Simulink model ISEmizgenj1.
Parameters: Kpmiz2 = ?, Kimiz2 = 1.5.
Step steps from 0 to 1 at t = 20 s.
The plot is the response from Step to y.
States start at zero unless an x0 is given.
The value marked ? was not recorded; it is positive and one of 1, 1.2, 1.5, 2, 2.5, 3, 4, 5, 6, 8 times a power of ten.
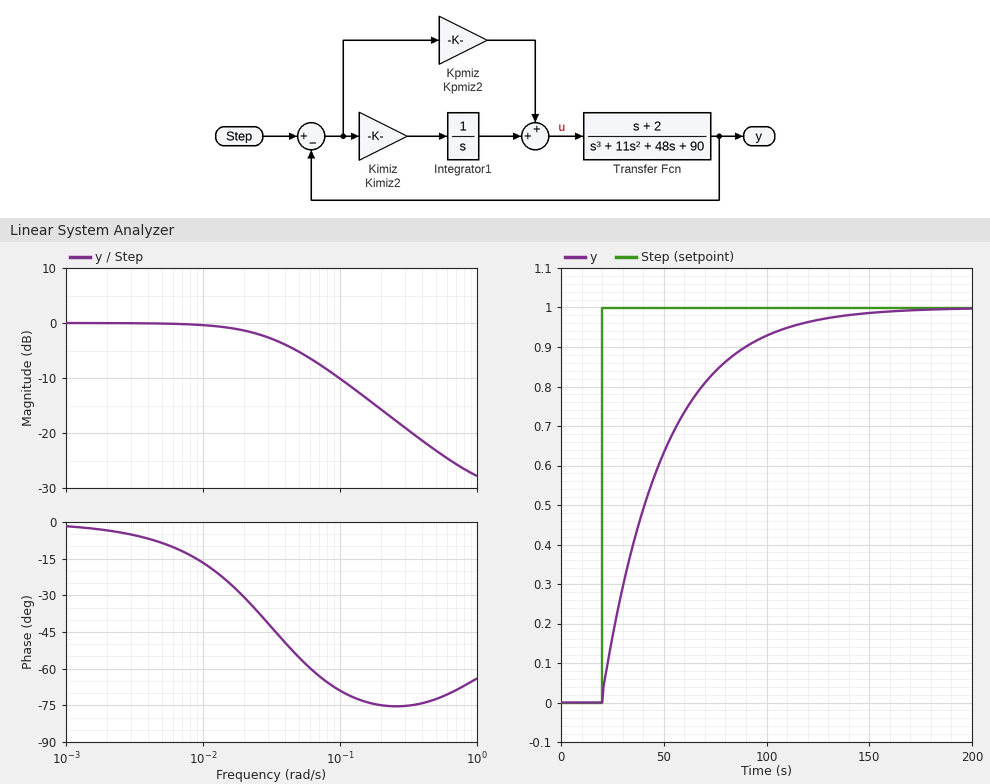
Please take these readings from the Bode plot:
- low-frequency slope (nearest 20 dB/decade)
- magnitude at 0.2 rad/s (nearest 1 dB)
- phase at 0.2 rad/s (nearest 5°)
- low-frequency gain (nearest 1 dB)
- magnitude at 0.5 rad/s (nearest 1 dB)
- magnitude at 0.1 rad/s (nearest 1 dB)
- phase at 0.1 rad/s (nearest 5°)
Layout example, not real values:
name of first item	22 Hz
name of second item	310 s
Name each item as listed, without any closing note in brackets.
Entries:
low-frequency slope	0 dB/decade
magnitude at 0.2 rad/s	-16 dB
phase at 0.2 rad/s	-75°
low-frequency gain	0 dB
magnitude at 0.5 rad/s	-23 dB
magnitude at 0.1 rad/s	-10 dB
phase at 0.1 rad/s	-70°
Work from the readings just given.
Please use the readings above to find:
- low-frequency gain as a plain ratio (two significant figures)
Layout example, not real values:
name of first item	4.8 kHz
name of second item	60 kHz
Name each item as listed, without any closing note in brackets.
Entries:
low-frequency gain as a plain ratio	1.0
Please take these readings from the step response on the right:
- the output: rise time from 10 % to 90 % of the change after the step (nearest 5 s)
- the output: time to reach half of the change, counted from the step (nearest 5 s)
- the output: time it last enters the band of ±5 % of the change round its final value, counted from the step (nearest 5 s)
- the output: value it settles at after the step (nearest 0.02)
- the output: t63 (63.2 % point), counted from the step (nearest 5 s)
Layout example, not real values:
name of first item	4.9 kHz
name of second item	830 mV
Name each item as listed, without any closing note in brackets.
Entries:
the output: rise time from 10 % to 90 % of the change after the step	65 s
the output: time to reach half of the change, counted from the step	20 s
the output: time it last enters the band of ±5 % of the change round its final value, counted from the step	90 s
the output: value it settles at after the step	1.00
the output: t63 (63.2 % point), counted from the step	30 s
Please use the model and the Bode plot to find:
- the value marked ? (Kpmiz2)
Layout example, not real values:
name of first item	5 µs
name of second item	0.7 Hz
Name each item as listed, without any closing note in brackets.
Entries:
the value marked ?	0.8
